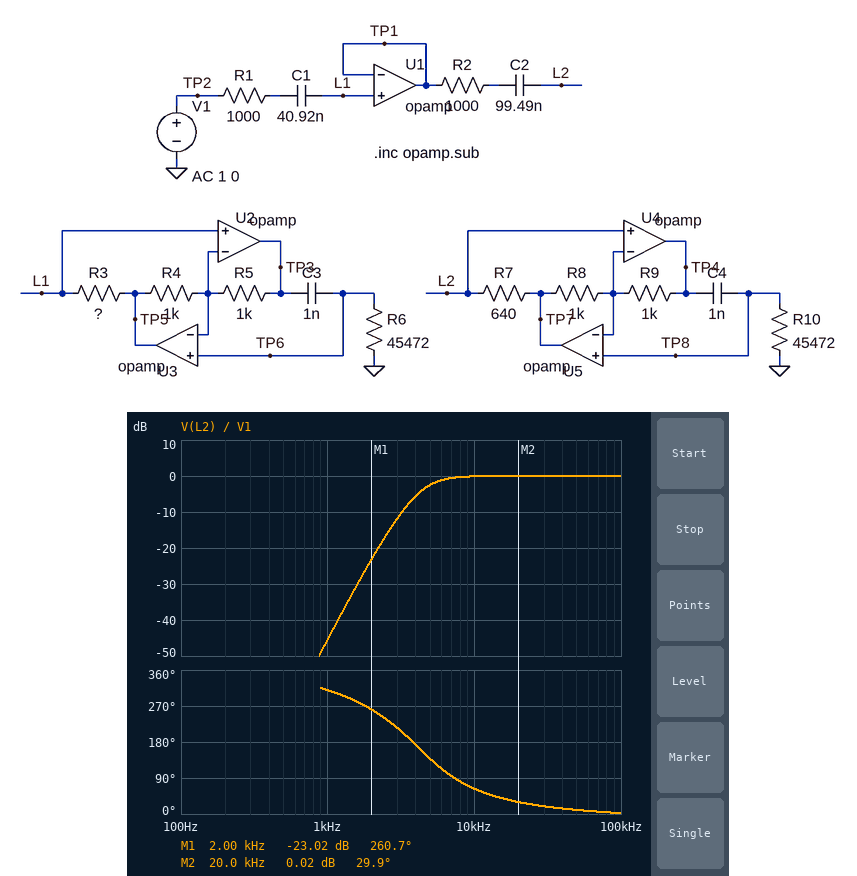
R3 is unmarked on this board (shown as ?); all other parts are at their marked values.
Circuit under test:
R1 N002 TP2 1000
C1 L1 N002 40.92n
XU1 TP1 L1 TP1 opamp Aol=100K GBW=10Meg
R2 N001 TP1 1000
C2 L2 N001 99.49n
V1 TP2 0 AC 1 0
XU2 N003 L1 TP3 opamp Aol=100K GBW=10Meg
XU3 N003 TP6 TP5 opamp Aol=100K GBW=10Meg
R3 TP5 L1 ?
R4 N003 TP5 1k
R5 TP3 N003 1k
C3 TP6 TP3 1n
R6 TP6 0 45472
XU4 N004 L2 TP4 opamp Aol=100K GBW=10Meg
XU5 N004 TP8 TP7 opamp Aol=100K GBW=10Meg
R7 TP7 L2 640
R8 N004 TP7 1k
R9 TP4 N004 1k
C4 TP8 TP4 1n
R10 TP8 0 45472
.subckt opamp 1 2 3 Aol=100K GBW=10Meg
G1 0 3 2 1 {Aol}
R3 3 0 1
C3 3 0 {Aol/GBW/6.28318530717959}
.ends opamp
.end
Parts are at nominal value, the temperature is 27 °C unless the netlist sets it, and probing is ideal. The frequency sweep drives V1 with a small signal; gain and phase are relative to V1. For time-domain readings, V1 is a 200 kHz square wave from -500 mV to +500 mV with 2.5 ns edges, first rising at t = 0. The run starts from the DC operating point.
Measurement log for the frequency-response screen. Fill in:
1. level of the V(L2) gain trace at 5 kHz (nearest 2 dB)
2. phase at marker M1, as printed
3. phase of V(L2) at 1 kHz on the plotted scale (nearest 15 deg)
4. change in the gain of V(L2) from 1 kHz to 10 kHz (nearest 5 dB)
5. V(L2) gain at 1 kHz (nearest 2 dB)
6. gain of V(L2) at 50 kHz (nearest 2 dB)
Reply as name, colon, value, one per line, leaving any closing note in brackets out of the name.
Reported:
level of the V(L2) gain trace at 5 kHz: -2 dB
phase at marker M1, as printed: 260.7 deg
phase of V(L2) at 1 kHz on the plotted scale: 315 deg
change in the gain of V(L2) from 1 kHz to 10 kHz: 45 dB
V(L2) gain at 1 kHz: -46 dB
gain of V(L2) at 50 kHz: 0 dB
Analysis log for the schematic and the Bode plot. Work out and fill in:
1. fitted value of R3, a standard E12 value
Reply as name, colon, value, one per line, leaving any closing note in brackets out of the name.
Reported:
fitted value of R3, a standard E12 value: 680 Ω
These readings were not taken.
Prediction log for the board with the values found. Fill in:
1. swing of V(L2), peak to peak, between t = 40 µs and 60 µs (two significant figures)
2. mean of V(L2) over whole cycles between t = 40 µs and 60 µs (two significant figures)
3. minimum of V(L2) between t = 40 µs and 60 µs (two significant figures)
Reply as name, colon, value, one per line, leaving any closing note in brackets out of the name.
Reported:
swing of V(L2), peak to peak, between t = 40 µs and 60 µs: 1.1 V
mean of V(L2) over whole cycles between t = 40 µs and 60 µs: -160 mV
minimum of V(L2) between t = 40 µs and 60 µs: -690 mV
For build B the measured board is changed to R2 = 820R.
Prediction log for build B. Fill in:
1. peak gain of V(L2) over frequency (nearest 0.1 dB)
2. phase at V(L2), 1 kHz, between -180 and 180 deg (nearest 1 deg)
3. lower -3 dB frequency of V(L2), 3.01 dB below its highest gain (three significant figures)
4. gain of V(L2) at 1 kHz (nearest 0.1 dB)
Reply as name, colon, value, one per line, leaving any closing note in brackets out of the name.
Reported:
peak gain of V(L2) over frequency: 0.3 dB
phase at V(L2), 1 kHz, between -180 and 180 deg: -45 deg
lower -3 dB frequency of V(L2), 3.01 dB below its highest gain: 4.37 kHz
gain of V(L2) at 1 kHz: -44.9 dB
